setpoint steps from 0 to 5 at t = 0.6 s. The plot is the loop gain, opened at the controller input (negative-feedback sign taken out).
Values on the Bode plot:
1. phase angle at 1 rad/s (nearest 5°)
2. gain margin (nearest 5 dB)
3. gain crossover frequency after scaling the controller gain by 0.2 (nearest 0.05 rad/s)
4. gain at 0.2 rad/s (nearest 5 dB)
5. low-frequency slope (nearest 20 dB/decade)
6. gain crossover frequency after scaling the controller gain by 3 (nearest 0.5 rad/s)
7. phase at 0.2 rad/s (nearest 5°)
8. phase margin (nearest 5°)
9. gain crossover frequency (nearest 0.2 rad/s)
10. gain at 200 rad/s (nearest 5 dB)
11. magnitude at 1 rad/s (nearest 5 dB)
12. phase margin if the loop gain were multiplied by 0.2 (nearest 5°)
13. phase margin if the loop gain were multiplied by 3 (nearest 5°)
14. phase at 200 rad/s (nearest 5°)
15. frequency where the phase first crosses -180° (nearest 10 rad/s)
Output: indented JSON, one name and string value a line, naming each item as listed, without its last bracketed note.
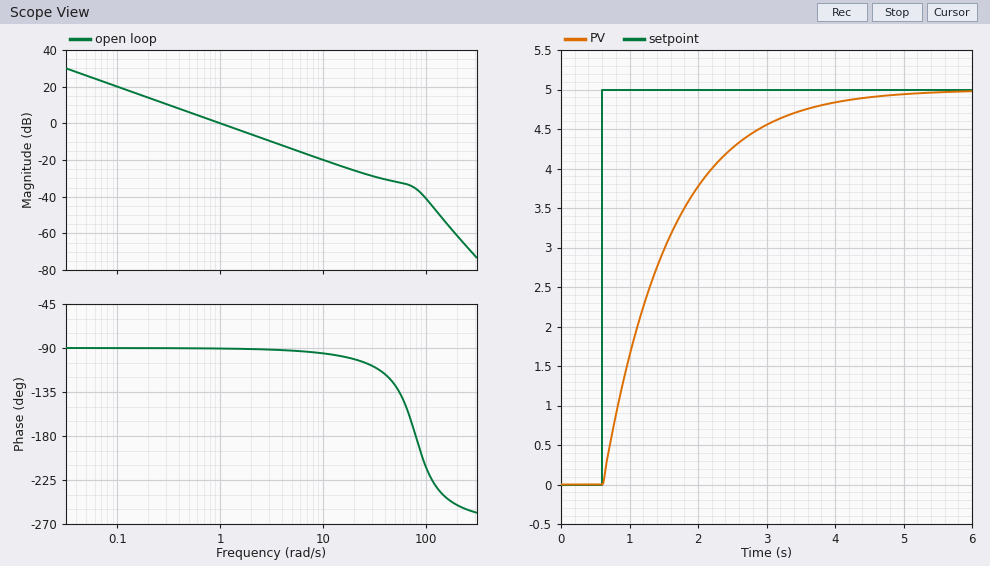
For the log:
{
  "phase angle at 1 rad/s": "-90°",
  "gain margin": "35 dB",
  "gain crossover frequency after scaling the controller gain by 0.2": "0.20 rad/s",
  "gain at 0.2 rad/s": "15 dB",
  "low-frequency slope": "-20 dB/decade",
  "gain crossover frequency after scaling the controller gain by 3": "3.0 rad/s",
  "phase at 0.2 rad/s": "-90°",
  "phase margin": "90°",
  "gain crossover frequency": "1.0 rad/s",
  "gain at 200 rad/s": "-60 dB",
  "magnitude at 1 rad/s": "0 dB",
  "phase margin if the loop gain were multiplied by 0.2": "90°",
  "phase margin if the loop gain were multiplied by 3": "90°",
  "phase at 200 rad/s": "-250°",
  "frequency where the phase first crosses -180°": "80 rad/s"
}
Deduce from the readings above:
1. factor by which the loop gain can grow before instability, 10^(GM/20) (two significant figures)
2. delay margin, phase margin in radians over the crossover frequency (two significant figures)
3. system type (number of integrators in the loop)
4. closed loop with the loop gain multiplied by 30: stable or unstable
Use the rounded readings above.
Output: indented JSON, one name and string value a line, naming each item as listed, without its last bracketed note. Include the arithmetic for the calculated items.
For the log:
{
  "factor by which the loop gain can grow before instability, 10^(GM/20)": "10^(35 / 20) = 56",
  "delay margin, phase margin in radians over the crossover frequency": "90 × π / 180 / 1 = 1.6 s",
  "system type": "1",
  "closed loop with the loop gain multiplied by 30: stable or unstable": "stable"
}
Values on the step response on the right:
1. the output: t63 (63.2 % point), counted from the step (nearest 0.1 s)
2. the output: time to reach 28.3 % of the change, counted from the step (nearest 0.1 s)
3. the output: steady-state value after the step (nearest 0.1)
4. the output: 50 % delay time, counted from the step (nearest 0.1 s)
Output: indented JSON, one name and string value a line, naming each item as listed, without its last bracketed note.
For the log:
{
  "the output: t63 (63.2 % point), counted from the step": "1.0 s",
  "the output: time to reach 28.3 % of the change, counted from the step": "0.3 s",
  "the output: steady-state value after the step": "5.0",
  "the output: 50 % delay time, counted from the step": "0.7 s"
}
